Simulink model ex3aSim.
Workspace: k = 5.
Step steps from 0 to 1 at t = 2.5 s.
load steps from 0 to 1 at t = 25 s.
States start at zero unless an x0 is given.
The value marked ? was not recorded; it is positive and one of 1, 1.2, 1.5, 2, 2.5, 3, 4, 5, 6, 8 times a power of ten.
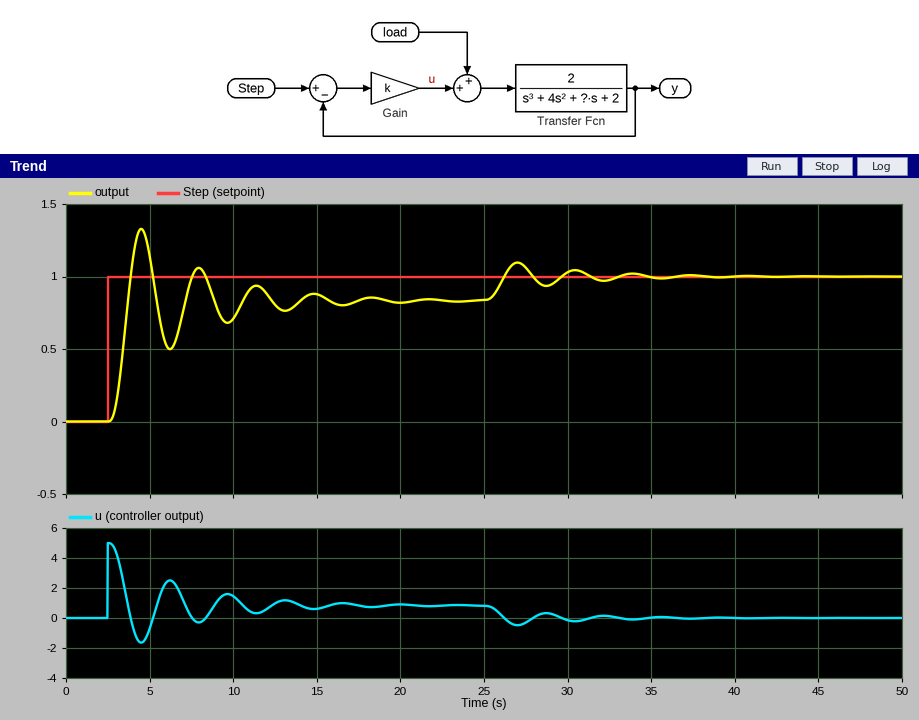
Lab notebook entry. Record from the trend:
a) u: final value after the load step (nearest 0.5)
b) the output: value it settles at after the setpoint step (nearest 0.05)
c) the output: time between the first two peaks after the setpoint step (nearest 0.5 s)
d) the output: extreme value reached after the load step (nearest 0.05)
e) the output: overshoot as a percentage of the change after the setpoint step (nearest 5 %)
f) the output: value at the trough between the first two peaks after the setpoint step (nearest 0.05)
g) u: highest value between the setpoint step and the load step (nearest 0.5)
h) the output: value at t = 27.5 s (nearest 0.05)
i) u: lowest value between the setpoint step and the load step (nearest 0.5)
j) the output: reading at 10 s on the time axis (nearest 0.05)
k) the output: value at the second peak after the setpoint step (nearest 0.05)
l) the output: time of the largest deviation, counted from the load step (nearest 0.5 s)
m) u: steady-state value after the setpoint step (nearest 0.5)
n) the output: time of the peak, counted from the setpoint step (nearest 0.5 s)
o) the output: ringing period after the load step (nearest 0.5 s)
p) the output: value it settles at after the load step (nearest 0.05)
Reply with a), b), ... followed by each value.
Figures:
a) 0.0
b) 0.85
c) 3.5 s
d) 1.10
e) 60 %
f) 0.50
g) 5.0
h) 1.05
i) -1.5
j) 0.70
k) 1.05
l) 2.0 s
m) 1.0
n) 2.0 s
o) 3.5 s
p) 1.00
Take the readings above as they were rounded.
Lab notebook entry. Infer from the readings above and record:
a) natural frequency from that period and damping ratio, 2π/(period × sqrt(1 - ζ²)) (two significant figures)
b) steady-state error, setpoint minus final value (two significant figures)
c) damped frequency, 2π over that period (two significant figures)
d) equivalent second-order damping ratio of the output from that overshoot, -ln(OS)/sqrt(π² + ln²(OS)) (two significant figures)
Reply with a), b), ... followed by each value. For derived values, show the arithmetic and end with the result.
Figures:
a) 2π / (3.5 × sqrt(1 - 0.16²)) = 1.8 rad/s
b) 1 - 0.85 = 0.15
c) 2π / 3.5 = 1.8 rad/s
d) ln(0.6) = -0.511; 0.511 / sqrt(9.870 + 0.261) = 0.16
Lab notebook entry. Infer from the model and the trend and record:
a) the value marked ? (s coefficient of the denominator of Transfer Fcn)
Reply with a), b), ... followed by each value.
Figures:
a) 5
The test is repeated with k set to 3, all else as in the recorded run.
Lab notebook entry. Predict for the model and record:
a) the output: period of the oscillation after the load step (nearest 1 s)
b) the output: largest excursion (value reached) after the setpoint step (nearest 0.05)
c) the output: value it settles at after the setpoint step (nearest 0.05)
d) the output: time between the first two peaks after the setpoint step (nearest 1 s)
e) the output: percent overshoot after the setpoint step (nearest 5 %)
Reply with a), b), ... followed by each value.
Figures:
a) 4 s
b) 1.05
c) 0.75
d) 4 s
e) 40 %
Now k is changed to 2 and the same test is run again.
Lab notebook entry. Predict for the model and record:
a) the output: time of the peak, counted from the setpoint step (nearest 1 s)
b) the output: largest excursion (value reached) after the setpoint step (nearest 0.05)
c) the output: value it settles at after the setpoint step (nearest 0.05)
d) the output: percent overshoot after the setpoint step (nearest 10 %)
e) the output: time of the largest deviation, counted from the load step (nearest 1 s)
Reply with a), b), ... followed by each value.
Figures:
a) 3 s
b) 0.85
c) 0.65
d) 30 %
e) 3 s
